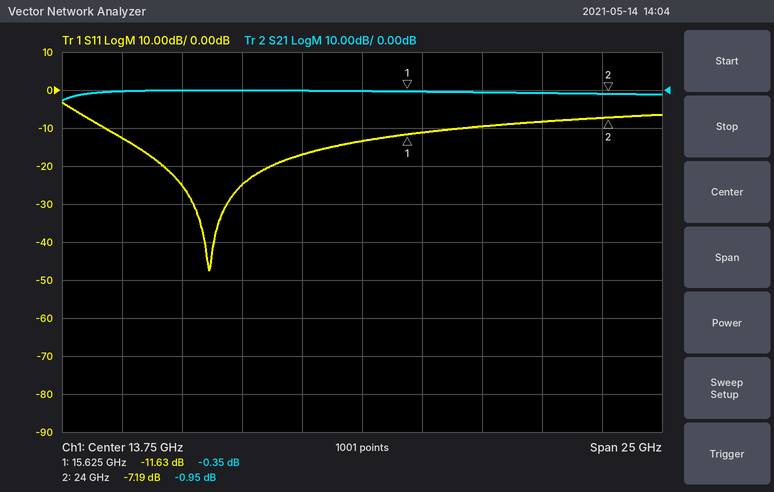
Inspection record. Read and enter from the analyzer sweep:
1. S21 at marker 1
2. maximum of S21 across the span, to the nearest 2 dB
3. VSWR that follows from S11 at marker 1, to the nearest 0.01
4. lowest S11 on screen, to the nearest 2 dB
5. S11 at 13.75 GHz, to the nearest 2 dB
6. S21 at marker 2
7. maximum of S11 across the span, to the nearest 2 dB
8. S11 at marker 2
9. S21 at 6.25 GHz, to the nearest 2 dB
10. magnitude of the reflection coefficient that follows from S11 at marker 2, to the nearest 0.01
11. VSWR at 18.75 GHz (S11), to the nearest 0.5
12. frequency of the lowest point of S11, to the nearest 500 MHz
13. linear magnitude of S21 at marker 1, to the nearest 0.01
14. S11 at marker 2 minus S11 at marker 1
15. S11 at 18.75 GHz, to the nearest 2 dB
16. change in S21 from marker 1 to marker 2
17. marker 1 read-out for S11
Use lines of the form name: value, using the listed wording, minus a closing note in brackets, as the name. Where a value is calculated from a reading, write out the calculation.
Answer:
S21 at marker 1: -0.35 dB
maximum of S21 across the span, to the nearest 2 dB: 0 dB
VSWR that follows from S11 at marker 1, to the nearest 0.01: (1 + 0.2621)/(1 − 0.2621) ≈ 1.71
lowest S11 on screen, to the nearest 2 dB: -48 dB
S11 at 13.75 GHz, to the nearest 2 dB: -14 dB
S21 at marker 2: -0.95 dB
maximum of S11 across the span, to the nearest 2 dB: -4 dB
S11 at marker 2: -7.19 dB
S21 at 6.25 GHz, to the nearest 2 dB: 0 dB
magnitude of the reflection coefficient that follows from S11 at marker 2, to the nearest 0.01: 10^(-7.19/20) ≈ 0.44
VSWR at 18.75 GHz (S11), to the nearest 0.5: |Γ| = 10^(-10/20) = 0.3162; VSWR = (1 + 0.3162)/(1 − 0.3162) ≈ 1.92, so 2.0 to the nearest 0.5
frequency of the lowest point of S11, to the nearest 500 MHz: 7.5 GHz
linear magnitude of S21 at marker 1, to the nearest 0.01: 10^(-0.35/20) ≈ 0.96
S11 at marker 2 minus S11 at marker 1: -7.19 − (-11.63) = 4.44 dB
S11 at 18.75 GHz, to the nearest 2 dB: -10 dB
change in S21 from marker 1 to marker 2: -0.95 − (-0.35) = -0.60 dB
marker 1 read-out for S11: -11.63 dB
